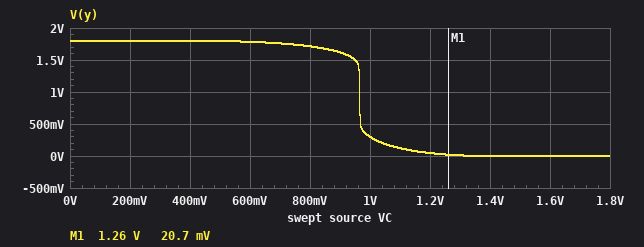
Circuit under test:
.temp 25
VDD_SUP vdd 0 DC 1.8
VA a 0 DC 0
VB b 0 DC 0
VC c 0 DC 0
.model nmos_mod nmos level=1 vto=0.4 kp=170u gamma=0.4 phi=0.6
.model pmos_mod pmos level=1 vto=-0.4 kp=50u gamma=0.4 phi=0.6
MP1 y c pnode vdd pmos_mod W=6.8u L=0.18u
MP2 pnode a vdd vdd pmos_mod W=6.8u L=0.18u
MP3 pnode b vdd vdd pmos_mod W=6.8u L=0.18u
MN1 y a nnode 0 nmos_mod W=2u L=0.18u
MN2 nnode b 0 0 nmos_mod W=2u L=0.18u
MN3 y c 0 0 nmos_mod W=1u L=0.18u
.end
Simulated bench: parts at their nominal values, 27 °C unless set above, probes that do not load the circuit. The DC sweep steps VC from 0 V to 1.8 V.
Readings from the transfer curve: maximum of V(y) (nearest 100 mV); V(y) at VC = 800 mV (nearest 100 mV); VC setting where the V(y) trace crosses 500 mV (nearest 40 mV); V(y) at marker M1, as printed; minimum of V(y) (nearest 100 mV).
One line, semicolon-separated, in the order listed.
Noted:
1.8 V; 1.7 V; 960 mV; 20.7 mV; 0 V
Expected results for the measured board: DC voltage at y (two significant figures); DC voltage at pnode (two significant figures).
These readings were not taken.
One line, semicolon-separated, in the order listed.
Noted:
1.8 V; 1.8 V
